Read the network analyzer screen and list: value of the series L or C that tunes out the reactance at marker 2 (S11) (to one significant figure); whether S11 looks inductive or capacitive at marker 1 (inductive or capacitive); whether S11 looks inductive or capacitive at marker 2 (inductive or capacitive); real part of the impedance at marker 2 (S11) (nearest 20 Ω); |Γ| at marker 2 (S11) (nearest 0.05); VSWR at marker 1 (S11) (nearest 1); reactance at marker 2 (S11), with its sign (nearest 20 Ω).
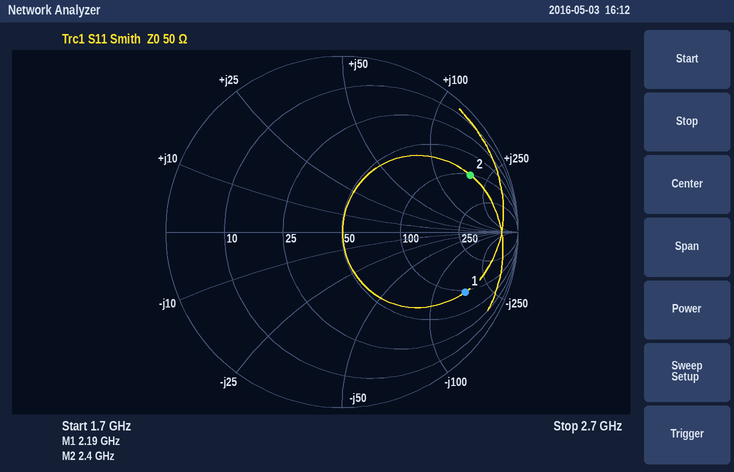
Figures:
400 fF
capacitive
inductive
100 Ω
0.80
8
+180 Ω
